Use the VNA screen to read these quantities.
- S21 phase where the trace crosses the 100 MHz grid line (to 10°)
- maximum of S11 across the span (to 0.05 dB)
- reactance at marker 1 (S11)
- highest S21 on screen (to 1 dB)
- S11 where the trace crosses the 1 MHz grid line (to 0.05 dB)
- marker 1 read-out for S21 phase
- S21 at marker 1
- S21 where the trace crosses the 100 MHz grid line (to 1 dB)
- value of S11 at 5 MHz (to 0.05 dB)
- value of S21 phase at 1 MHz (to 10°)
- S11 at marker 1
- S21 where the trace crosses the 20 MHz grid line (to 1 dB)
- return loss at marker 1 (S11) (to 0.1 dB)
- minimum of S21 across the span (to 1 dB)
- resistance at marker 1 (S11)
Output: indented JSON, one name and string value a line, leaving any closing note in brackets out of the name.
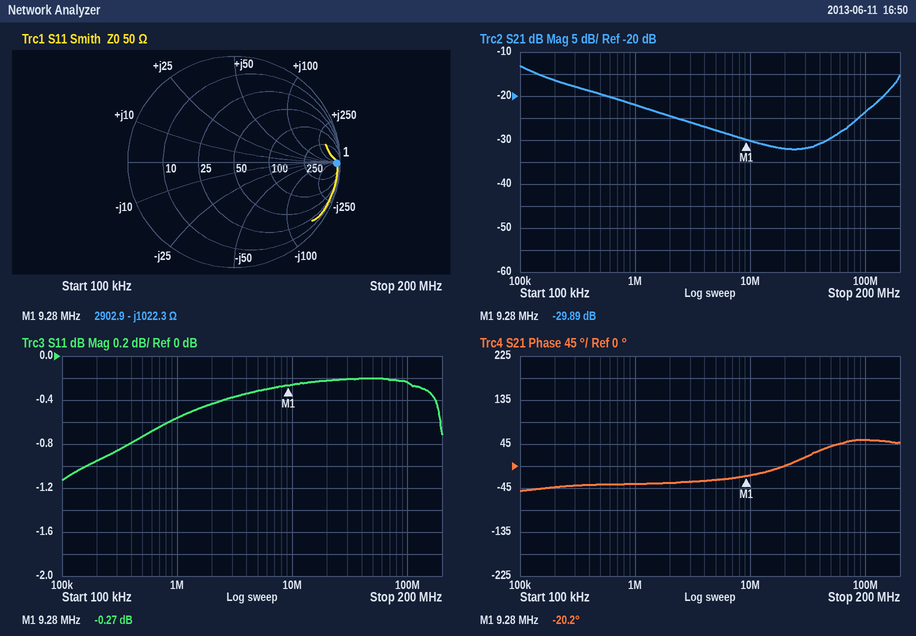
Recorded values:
{
  "S21 phase where the trace crosses the 100 MHz grid line": "50°",
  "maximum of S11 across the span": "-0.20 dB",
  "reactance at marker 1": "-1022.3 Ω",
  "highest S21 on screen": "-13 dB",
  "S11 where the trace crosses the 1 MHz grid line": "-0.55 dB",
  "marker 1 read-out for S21 phase": "-20.2°",
  "S21 at marker 1": "-29.89 dB",
  "S21 where the trace crosses the 100 MHz grid line": "-24 dB",
  "value of S11 at 5 MHz": "-0.30 dB",
  "value of S21 phase at 1 MHz": "-40°",
  "S11 at marker 1": "-0.27 dB",
  "S21 where the trace crosses the 20 MHz grid line": "-32 dB",
  "return loss at marker 1 (S11)": "0.3 dB",
  "minimum of S21 across the span": "-32 dB",
  "resistance at marker 1": "2902.9 Ω"
}
